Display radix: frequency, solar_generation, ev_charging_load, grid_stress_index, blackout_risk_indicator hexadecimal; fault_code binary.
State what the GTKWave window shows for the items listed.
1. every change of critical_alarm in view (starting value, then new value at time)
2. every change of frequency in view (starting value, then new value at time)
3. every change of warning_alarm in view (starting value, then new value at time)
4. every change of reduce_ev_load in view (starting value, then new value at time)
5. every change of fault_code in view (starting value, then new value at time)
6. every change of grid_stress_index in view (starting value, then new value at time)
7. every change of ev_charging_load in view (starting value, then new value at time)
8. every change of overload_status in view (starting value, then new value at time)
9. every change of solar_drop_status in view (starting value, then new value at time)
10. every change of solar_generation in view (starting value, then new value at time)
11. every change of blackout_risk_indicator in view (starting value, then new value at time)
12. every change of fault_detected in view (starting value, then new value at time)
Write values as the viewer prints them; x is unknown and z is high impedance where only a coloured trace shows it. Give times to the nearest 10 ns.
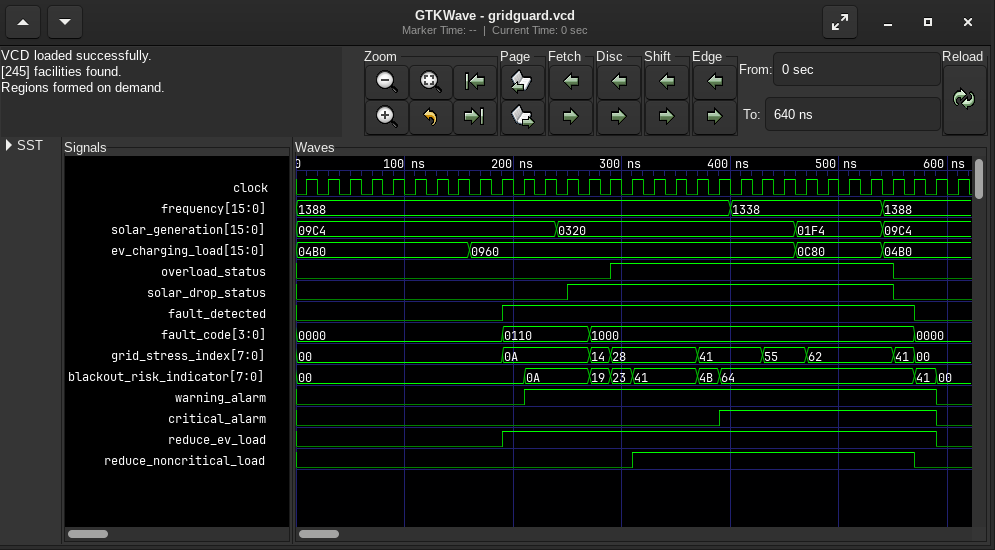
0, 1 at 390 ns, 0 at 590 ns
1388, 1338 at 400 ns, 1388 at 540 ns
0, 1 at 210 ns, 0 at 590 ns
0, 1 at 190 ns, 0 at 590 ns
0000, 0110 at 190 ns, 1000 at 270 ns, 0000 at 570 ns
00, 0A at 190 ns, 14 at 270 ns, 28 at 290 ns, 41 at 370 ns, 55 at 430 ns, 62 at 470 ns, 41 at 550 ns, 00 at 570 ns
04B0, 0960 at 160 ns, 0C80 at 460 ns, 04B0 at 540 ns
0, 1 at 290 ns, 0 at 550 ns
0, 1 at 250 ns, 0 at 550 ns
09C4, 0320 at 240 ns, 01F4 at 460 ns, 09C4 at 540 ns
00, 0A at 210 ns, 19 at 270 ns, 23 at 290 ns, 41 at 310 ns, 4B at 370 ns, 64 at 390 ns, 41 at 570 ns, 00 at 590 ns
0, 1 at 190 ns, 0 at 570 ns
